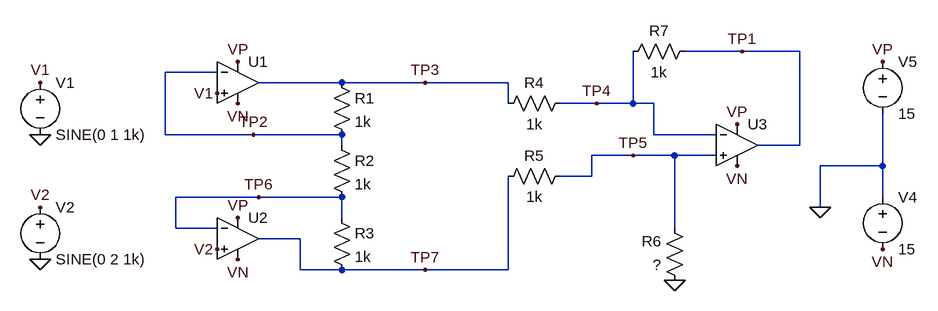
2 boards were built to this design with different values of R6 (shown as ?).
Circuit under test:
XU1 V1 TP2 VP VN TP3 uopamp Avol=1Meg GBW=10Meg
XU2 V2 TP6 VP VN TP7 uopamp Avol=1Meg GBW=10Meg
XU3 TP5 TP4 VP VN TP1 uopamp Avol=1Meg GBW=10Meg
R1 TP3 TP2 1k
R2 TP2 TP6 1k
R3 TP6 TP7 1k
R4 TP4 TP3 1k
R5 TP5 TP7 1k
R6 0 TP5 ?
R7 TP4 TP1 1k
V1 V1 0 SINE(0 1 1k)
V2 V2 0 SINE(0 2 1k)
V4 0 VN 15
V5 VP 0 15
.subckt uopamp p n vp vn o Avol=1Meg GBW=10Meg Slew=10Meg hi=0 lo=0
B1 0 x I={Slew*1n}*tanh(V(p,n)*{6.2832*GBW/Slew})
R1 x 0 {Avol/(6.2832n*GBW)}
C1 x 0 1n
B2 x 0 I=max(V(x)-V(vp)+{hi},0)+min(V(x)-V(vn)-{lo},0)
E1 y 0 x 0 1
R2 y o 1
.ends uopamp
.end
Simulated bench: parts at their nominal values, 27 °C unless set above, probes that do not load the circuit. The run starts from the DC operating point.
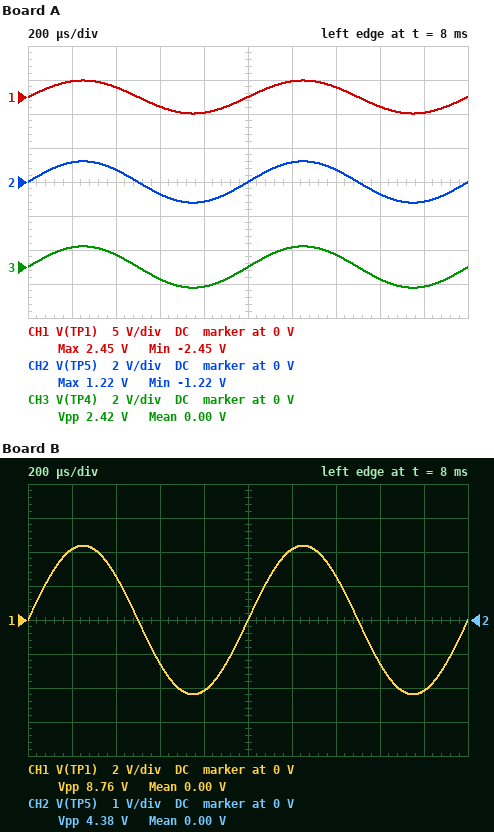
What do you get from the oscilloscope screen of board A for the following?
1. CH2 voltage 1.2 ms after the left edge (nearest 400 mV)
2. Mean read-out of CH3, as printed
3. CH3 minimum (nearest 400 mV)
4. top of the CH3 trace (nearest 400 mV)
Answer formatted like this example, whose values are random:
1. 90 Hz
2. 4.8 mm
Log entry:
1. 1.2 V
2. 0.00 V
3. -1.2 V
4. 1.2 V
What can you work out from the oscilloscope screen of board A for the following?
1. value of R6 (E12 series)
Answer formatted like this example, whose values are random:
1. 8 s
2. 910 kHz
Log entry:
1. 680 Ω
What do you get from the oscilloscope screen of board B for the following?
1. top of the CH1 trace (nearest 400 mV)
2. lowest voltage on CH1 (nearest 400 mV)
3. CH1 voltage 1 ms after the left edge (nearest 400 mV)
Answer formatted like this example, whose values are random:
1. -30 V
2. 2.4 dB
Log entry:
1. 4.4 V
2. -4.4 V
3. 0 V
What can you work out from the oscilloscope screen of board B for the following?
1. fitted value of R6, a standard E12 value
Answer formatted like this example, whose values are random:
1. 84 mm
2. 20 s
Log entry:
1. 2.7 kΩ
